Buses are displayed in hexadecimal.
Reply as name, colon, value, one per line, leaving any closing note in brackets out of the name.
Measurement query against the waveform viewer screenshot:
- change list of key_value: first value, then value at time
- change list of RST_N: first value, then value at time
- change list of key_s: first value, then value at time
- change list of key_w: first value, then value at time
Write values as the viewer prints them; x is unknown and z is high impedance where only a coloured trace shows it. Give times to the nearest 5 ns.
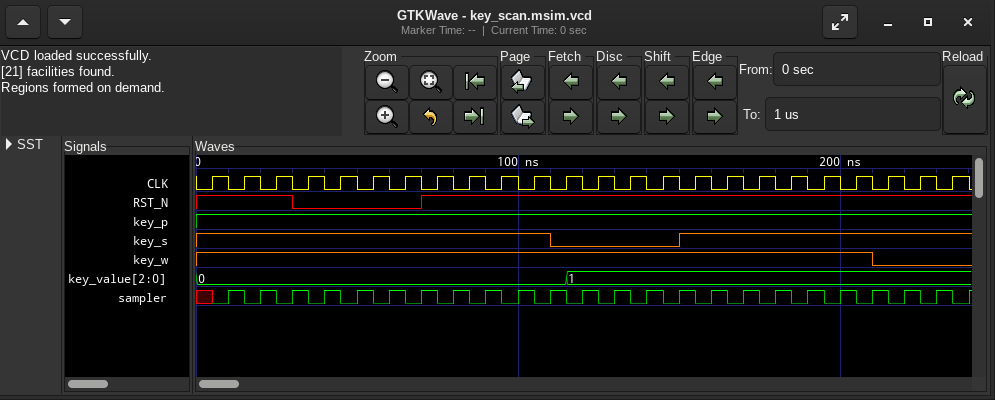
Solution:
change list of key_value: first value, then value at time: 0, 1 at 115 ns
change list of RST_N: first value, then value at time: 1, 0 at 30 ns, 1 at 70 ns
change list of key_s: first value, then value at time: 1, 0 at 110 ns, 1 at 150 ns
change list of key_w: first value, then value at time: 1, 0 at 210 ns
